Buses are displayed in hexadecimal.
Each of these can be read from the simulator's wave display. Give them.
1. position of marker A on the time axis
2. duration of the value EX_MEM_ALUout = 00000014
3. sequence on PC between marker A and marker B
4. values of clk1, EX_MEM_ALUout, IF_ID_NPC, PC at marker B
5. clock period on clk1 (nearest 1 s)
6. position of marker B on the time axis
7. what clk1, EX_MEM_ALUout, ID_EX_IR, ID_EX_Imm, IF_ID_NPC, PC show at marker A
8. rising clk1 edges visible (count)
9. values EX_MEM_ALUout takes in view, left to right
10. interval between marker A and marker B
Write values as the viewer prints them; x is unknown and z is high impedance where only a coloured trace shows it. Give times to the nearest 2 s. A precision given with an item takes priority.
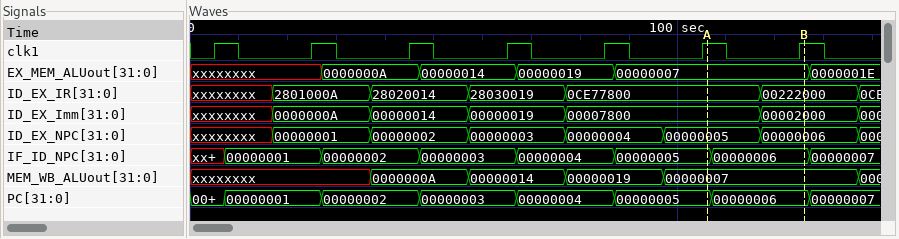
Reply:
106 s
20 s
00000005, 00000006
clk1=1, EX_MEM_ALUout=00000007, IF_ID_NPC=00000006, PC=00000006
20 s
126 s
clk1=1, EX_MEM_ALUout=00000007, ID_EX_IR=0CE77800, ID_EX_Imm=00007800, IF_ID_NPC=00000005, PC=00000005
7
xxxxxxxx, 0000000A, 00000014, 00000019, 00000007, 0000001E
20 s
